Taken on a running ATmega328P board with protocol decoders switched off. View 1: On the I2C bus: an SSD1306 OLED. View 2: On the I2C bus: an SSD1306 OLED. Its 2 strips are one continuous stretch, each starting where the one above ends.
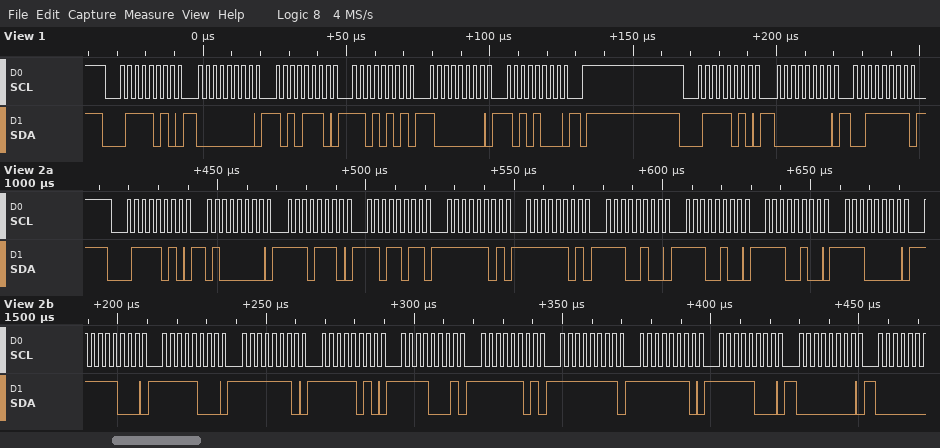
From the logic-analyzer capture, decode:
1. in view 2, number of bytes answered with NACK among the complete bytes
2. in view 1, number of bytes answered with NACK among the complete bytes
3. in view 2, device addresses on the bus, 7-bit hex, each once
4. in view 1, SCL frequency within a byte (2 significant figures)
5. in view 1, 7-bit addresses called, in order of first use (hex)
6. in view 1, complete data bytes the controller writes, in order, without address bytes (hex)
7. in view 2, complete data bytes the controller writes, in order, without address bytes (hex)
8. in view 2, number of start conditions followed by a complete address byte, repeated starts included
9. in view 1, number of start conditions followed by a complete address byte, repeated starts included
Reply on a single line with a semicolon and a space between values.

0; 0; 0x3D; 400 kHz; 0x3D; 00 AE D5 80 A8 00 3F; 40 EE DB FD FD E4 E4 E4 E0 F8 F8 FE FA F1 FD FF FE F8 00; 1; 2
